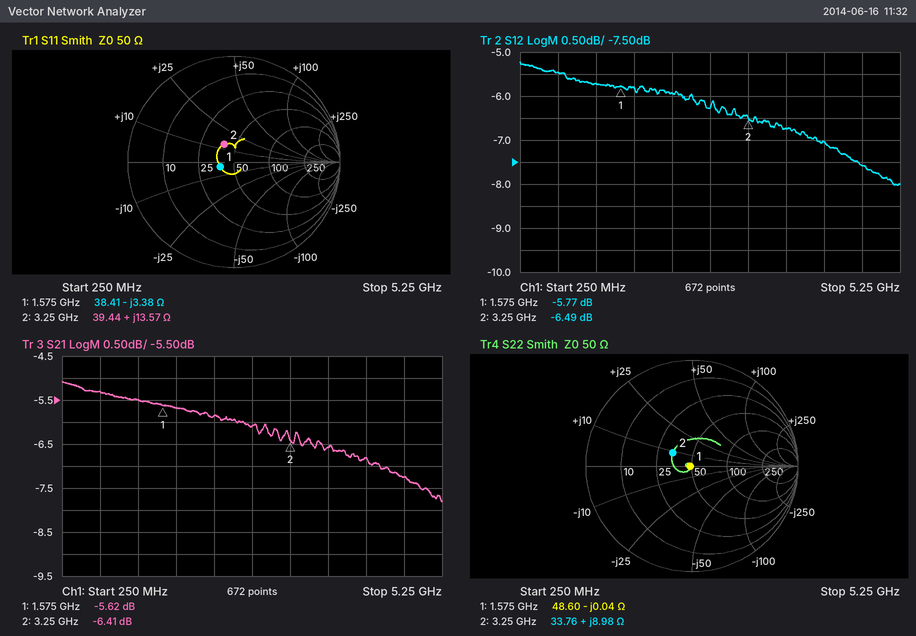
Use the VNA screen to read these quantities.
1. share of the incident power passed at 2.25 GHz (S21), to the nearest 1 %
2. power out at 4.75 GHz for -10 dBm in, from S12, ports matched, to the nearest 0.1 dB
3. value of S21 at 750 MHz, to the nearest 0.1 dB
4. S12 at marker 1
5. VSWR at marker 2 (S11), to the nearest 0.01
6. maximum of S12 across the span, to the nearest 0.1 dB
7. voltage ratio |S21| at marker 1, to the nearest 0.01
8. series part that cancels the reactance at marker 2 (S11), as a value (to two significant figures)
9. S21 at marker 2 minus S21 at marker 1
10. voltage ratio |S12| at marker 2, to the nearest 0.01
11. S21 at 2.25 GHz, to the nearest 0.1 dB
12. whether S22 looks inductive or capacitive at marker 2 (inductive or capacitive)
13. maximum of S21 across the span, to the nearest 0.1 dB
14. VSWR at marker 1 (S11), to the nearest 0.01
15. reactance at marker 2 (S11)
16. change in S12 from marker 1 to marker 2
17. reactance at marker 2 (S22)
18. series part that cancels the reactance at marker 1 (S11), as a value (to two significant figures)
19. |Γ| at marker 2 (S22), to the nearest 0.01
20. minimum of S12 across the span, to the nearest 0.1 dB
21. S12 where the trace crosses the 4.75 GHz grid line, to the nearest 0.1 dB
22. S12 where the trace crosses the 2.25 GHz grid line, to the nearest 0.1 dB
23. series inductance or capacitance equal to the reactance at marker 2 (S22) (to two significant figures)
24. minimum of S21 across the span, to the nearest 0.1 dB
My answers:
26 %
-17.6 dBm
-5.3 dB
-5.77 dB
1.47
-5.2 dB
0.52
3.6 pF
-0.79 dB
0.47
-5.9 dB
inductive
-5.1 dB
1.32
+13.57 Ω
-0.72 dB
+8.98 Ω
340 pH
0.22
-8.0 dB
-7.6 dB
-5.9 dB
440 pH
-7.8 dB
